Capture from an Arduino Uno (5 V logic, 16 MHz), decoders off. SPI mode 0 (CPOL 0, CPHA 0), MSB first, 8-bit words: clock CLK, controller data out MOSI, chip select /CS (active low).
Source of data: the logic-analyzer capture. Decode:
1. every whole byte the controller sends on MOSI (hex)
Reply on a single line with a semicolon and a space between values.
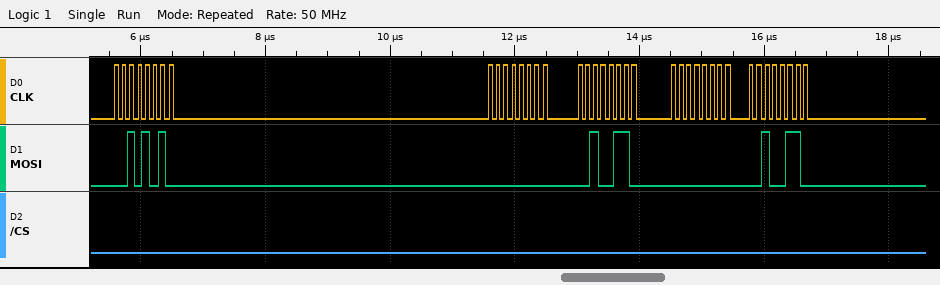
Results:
2A 00 26 00 26
